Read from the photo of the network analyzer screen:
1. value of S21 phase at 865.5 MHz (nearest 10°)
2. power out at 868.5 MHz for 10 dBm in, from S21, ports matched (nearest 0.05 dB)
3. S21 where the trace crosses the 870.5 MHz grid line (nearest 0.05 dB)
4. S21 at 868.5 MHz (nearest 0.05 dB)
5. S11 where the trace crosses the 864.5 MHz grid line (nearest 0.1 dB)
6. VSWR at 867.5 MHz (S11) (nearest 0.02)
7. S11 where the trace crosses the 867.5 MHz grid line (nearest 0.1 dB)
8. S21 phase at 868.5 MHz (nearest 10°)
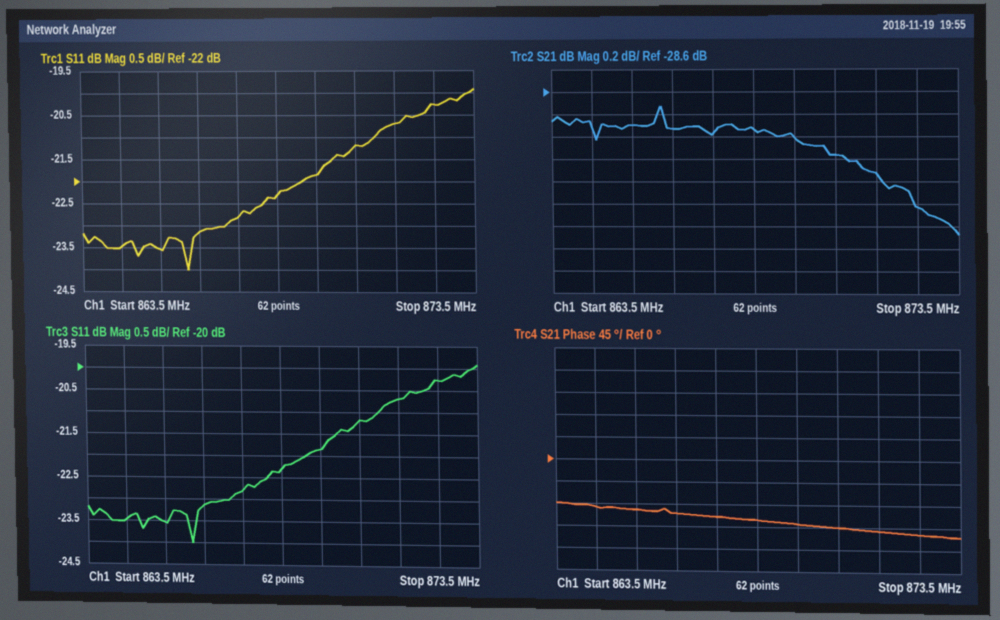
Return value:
-100°
-18.95 dBm
-29.15 dB
-28.95 dB
-23.5 dB
1.16
-22.8 dB
-120°
